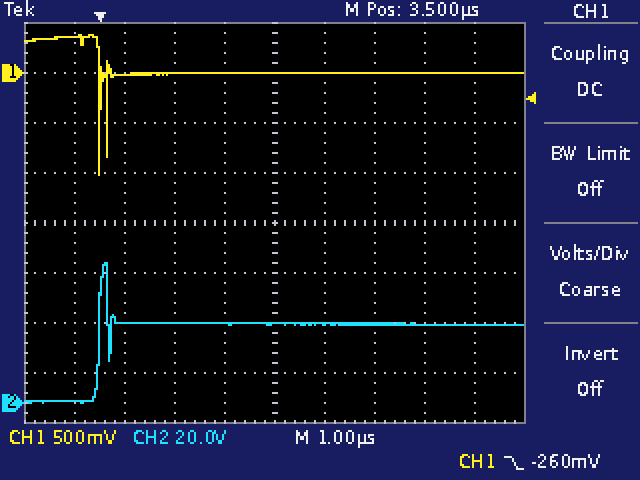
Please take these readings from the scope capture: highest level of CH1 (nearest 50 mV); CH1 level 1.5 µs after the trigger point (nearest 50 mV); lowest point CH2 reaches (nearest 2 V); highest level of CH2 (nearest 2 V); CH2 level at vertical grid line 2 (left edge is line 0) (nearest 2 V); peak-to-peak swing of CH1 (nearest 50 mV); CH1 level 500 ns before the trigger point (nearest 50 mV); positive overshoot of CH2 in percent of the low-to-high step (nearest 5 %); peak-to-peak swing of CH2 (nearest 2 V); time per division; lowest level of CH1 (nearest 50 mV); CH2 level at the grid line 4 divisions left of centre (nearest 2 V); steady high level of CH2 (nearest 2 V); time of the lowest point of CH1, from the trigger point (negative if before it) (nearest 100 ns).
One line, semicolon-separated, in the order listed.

400 mV; 0 mV; 0 V; 56 V; 32 V; 1.40 V; 350 mV; 80 %; 56 V; 1 µs; -1.00 V; 0 V; 32 V; 0.0 µs
